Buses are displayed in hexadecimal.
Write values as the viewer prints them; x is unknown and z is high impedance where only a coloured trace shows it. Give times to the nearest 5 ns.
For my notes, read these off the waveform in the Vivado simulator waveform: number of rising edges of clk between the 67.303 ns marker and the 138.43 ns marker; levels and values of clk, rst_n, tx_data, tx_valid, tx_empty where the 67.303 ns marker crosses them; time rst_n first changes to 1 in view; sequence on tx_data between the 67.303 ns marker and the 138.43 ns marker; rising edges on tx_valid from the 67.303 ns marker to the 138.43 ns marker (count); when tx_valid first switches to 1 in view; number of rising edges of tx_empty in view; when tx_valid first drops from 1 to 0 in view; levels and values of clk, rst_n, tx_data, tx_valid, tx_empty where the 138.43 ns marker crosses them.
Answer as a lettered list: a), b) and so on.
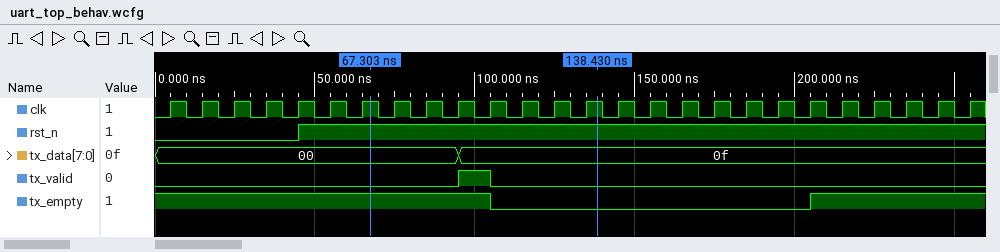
a) 7
b) clk=1, rst_n=1, tx_data=00, tx_valid=0, tx_empty=1
c) 45 ns
d) 00, 0f
e) 1
f) 95 ns
g) 1
h) 105 ns
i) clk=1, rst_n=1, tx_data=0f, tx_valid=0, tx_empty=0
